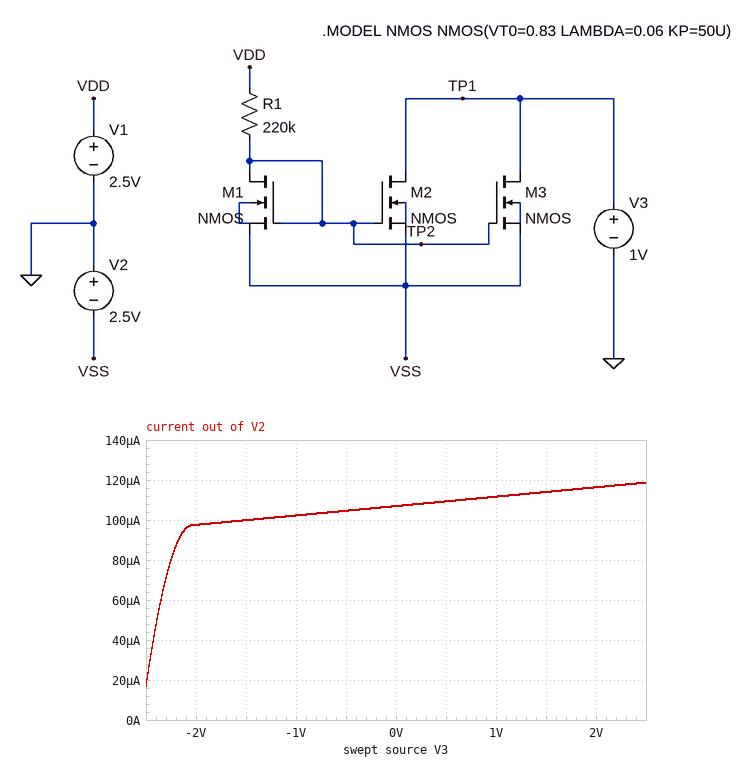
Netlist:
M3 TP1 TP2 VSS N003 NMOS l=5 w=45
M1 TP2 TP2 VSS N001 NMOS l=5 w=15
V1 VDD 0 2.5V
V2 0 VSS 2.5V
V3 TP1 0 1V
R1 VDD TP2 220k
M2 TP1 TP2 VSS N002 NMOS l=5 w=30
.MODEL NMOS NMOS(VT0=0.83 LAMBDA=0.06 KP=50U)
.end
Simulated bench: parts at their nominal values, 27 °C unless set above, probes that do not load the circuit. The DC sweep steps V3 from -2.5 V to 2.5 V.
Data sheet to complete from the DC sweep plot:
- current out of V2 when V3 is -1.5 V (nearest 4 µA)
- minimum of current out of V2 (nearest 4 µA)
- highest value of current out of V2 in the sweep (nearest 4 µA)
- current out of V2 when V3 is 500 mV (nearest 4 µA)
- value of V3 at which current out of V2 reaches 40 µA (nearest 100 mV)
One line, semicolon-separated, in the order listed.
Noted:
100 µA; 16 µA; 120 µA; 108 µA; -2.4 V
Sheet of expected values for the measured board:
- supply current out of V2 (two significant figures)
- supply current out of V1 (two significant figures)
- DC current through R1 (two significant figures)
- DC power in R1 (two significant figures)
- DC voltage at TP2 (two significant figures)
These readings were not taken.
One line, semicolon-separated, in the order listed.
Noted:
110 µA; 17 µA; 17 µA; 63 µW; -1.2 V
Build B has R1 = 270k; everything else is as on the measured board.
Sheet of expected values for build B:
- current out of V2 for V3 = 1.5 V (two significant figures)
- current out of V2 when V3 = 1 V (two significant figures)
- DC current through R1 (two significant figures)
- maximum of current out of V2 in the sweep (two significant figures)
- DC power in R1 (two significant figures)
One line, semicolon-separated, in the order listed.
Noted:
94 µA; 92 µA; 14 µA; 98 µA; 52 µW
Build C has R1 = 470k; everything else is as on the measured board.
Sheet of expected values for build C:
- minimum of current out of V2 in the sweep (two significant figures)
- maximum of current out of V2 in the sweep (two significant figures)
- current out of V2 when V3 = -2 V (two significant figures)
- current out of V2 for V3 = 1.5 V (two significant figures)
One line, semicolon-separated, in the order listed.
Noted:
8.2 µA; 58 µA; 48 µA; 56 µA
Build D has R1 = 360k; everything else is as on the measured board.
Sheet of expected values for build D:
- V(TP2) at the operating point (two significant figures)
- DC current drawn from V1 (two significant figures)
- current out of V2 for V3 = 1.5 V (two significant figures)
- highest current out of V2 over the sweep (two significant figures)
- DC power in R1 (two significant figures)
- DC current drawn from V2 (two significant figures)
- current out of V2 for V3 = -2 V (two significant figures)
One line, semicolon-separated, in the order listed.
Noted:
-1.3 V; 11 µA; 72 µA; 75 µA; 40 µW; 70 µA; 61 µA
